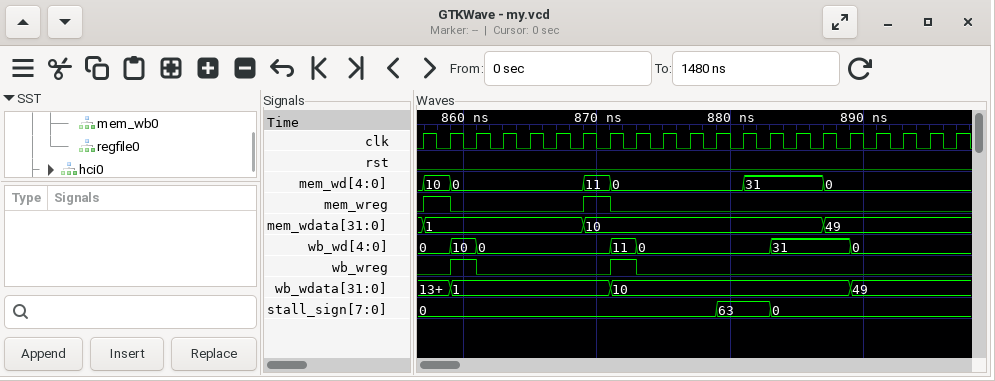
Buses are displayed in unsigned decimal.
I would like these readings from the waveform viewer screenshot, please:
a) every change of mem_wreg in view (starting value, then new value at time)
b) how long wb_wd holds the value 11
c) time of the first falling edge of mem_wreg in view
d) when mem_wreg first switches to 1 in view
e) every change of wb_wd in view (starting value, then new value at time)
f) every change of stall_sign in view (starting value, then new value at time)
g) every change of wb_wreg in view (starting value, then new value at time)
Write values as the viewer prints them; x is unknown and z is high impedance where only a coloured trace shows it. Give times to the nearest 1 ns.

0, 1 at 857 ns, 0 at 859 ns, 1 at 869 ns, 0 at 871 ns
2 ns
859 ns
857 ns
0, 10 at 859 ns, 0 at 861 ns, 11 at 871 ns, 0 at 873 ns, 31 at 883 ns, 0 at 889 ns
0, 63 at 879 ns, 0 at 883 ns
0, 1 at 859 ns, 0 at 861 ns, 1 at 871 ns, 0 at 873 ns
